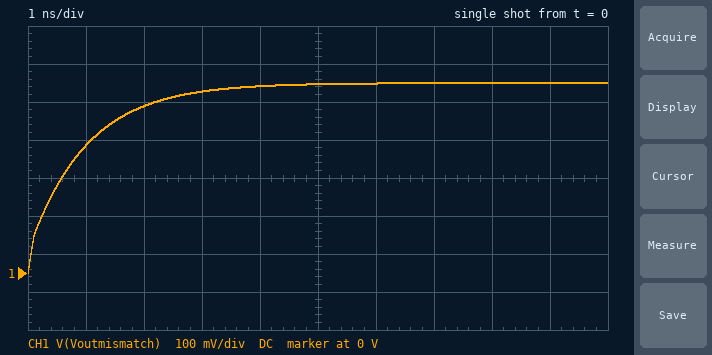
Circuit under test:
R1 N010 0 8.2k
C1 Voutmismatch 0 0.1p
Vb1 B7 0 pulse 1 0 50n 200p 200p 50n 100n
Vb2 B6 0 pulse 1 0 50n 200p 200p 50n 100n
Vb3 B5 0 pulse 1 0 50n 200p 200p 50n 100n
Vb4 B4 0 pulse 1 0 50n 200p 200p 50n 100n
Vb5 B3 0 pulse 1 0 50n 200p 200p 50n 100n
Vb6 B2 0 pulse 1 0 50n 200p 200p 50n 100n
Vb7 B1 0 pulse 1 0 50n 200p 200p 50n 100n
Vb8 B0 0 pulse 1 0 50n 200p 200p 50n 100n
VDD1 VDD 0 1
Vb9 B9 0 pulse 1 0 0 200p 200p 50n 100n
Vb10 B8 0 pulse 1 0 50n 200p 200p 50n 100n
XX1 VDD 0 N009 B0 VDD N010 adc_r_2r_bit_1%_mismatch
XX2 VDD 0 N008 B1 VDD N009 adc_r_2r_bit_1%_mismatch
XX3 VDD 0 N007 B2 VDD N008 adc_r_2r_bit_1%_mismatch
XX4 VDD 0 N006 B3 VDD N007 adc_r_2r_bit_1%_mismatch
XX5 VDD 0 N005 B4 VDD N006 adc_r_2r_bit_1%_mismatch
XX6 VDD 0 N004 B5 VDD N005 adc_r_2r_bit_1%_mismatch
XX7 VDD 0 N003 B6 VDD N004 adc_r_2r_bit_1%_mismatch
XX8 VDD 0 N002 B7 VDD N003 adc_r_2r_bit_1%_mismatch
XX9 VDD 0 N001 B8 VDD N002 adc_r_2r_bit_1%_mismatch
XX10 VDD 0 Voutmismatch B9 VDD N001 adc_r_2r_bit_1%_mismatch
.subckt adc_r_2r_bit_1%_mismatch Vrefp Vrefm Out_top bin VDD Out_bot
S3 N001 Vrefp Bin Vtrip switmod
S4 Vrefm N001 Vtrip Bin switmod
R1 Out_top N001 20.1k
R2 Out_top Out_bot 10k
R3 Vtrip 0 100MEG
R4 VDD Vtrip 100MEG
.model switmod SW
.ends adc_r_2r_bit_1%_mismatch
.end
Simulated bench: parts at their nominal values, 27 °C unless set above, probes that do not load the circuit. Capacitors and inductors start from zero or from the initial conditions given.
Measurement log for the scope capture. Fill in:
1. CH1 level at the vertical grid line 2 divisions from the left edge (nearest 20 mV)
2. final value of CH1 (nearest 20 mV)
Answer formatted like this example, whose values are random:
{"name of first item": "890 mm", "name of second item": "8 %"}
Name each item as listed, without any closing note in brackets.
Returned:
{"CH1 level at the vertical grid line 2 divisions from the left edge": "440 mV", "final value of CH1": "500 mV"}
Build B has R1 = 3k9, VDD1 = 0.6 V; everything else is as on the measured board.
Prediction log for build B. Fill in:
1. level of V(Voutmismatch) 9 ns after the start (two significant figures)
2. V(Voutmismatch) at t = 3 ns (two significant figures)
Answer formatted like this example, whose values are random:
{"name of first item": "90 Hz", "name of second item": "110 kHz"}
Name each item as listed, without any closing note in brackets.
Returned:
{"level of V(Voutmismatch) 9 ns after the start": "300 mV", "V(Voutmismatch) at t = 3 ns": "290 mV"}
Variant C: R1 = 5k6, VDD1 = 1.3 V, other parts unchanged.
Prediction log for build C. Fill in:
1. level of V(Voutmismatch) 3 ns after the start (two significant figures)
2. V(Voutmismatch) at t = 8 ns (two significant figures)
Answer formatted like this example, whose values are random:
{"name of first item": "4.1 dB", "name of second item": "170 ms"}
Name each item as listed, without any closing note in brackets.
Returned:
{"level of V(Voutmismatch) 3 ns after the start": "620 mV", "V(Voutmismatch) at t = 8 ns": "650 mV"}
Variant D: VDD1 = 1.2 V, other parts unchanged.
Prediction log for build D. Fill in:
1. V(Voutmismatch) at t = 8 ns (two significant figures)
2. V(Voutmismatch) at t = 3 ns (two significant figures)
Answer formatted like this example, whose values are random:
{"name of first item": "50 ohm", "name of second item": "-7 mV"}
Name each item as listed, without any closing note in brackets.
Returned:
{"V(Voutmismatch) at t = 8 ns": "600 mV", "V(Voutmismatch) at t = 3 ns": "570 mV"}
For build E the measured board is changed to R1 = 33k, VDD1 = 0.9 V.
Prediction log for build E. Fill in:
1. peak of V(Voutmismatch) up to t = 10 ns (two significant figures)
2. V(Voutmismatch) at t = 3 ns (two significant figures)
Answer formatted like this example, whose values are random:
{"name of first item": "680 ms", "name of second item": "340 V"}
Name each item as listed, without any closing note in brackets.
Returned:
{"peak of V(Voutmismatch) up to t = 10 ns": "450 mV", "V(Voutmismatch) at t = 3 ns": "430 mV"}
